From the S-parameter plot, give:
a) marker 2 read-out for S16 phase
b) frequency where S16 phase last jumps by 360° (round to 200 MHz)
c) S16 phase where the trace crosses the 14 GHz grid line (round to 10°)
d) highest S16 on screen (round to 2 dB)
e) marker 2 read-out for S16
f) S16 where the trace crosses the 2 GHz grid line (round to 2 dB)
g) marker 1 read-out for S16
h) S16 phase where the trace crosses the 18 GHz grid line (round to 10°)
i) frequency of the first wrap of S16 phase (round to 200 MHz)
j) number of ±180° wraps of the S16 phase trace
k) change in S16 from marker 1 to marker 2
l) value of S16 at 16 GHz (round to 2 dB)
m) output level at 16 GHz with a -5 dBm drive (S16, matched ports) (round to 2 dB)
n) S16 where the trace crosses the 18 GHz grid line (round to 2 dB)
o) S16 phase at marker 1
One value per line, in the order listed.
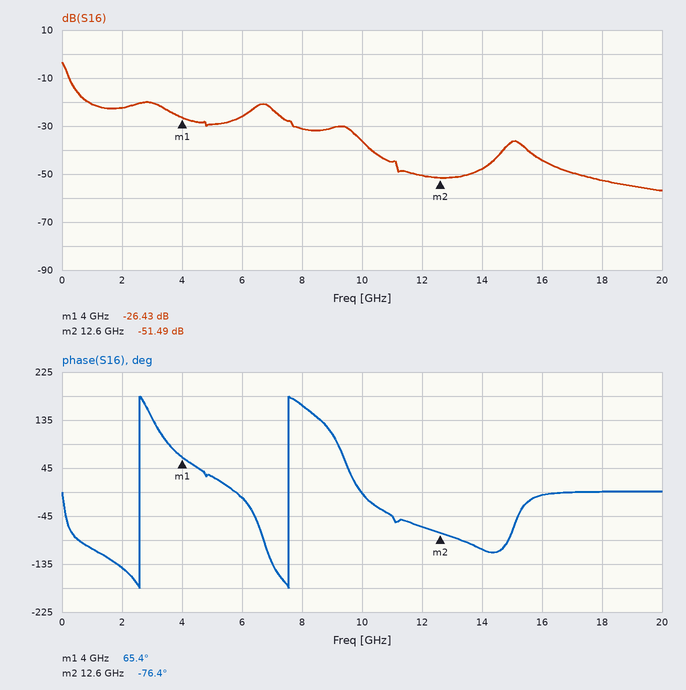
-76.4°
7.6 GHz
-110°
-4 dB
-51.49 dB
-22 dB
-26.43 dB
0°
2.6 GHz
2
-25.06 dB
-44 dB
-50 dBm
-52 dB
65.4°
